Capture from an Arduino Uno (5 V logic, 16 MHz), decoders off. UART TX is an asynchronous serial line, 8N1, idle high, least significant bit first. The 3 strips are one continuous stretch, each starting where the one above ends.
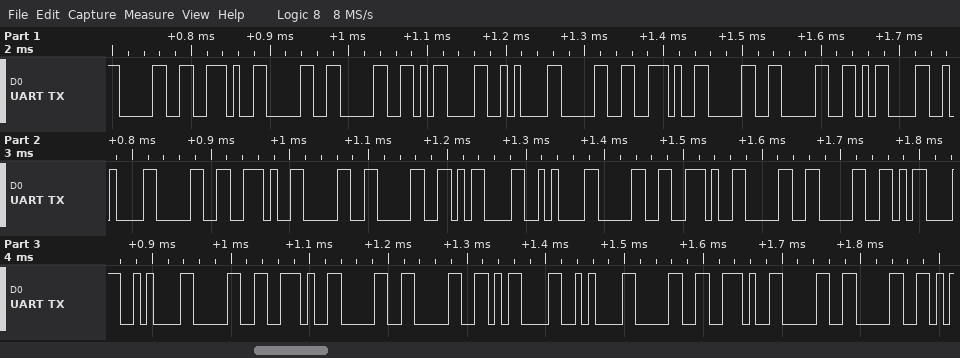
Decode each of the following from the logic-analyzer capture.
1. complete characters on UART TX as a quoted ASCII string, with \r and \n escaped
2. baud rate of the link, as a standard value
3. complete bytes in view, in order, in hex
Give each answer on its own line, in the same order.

"0.00\r\n0.00\r\n0.00\r\n0.00\r\n0.00\r\n0.00"
115200 baud
30 2E 30 30 0D 0A 30 2E 30 30 0D 0A 30 2E 30 30 0D 0A 30 2E 30 30 0D 0A 30 2E 30 30 0D 0A 30 2E 30 30
